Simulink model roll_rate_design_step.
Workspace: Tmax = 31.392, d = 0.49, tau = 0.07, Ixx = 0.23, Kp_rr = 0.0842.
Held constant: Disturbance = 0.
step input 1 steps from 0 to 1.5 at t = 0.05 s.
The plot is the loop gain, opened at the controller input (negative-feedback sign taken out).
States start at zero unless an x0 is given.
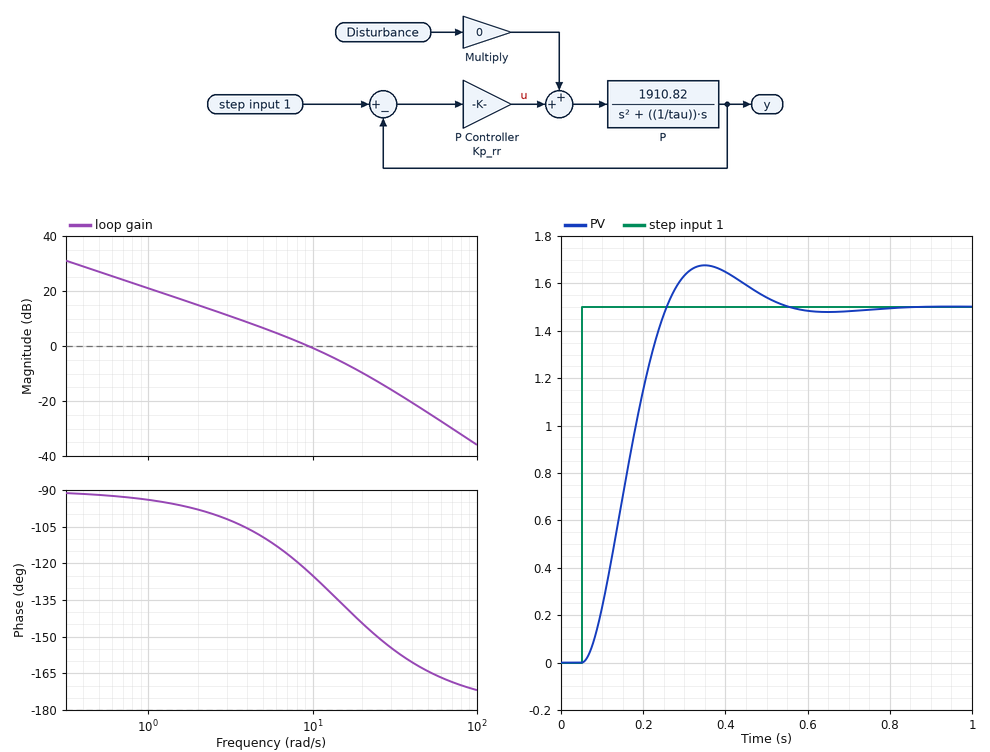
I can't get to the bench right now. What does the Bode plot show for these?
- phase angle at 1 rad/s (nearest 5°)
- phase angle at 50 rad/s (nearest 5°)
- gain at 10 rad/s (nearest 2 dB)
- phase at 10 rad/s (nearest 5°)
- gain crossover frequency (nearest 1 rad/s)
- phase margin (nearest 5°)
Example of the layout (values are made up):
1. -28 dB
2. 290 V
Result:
1. -95°
2. -165°
3. 0 dB
4. -125°
5. 9 rad/s
6. 55°
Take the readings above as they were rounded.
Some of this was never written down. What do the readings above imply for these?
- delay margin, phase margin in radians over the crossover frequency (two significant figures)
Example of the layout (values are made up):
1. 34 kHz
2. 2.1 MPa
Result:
1. 0.11 s
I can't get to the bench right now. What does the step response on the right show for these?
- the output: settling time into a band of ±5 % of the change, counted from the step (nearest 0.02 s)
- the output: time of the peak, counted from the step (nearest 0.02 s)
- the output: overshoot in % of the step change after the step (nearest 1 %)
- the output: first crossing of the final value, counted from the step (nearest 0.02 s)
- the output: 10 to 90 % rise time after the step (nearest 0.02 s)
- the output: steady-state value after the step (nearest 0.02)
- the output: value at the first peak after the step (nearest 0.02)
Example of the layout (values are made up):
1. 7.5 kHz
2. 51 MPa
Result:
1. 0.42 s
2. 0.30 s
3. 12 %
4. 0.20 s
5. 0.14 s
6. 1.50
7. 1.68
